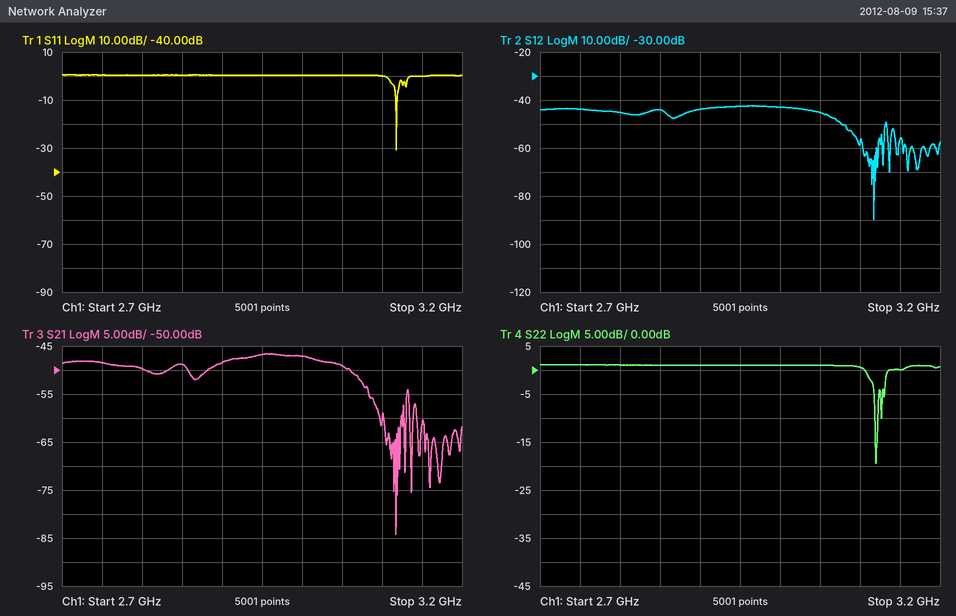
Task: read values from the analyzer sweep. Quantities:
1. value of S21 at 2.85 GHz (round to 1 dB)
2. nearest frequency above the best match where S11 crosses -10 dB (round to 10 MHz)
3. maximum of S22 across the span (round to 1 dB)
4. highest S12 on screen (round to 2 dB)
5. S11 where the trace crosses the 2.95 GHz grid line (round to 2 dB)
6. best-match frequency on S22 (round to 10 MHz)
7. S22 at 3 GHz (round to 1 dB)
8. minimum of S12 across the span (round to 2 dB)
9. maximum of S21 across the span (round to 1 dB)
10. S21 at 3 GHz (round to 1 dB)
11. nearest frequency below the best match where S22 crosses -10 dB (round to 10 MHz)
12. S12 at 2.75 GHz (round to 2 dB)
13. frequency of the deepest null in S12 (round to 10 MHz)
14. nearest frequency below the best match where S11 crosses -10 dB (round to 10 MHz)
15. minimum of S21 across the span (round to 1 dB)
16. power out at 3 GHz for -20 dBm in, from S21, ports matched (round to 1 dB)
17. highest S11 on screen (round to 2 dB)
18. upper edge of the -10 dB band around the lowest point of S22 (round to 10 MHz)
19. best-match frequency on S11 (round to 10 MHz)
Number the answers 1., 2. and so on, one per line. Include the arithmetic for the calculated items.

1. -49 dB
2. 3.12 GHz
3. 1 dB
4. -42 dB
5. 0 dB
6. 3.12 GHz
7. 1 dB
8. -90 dB
9. -47 dB
10. -47 dB
11. 3.12 GHz
12. -44 dB
13. 3.12 GHz
14. 3.12 GHz
15. -84 dB
16. -20 dBm + (-47 dB) = -67 dBm
17. 0 dB
18. 3.12 GHz
19. 3.12 GHz
